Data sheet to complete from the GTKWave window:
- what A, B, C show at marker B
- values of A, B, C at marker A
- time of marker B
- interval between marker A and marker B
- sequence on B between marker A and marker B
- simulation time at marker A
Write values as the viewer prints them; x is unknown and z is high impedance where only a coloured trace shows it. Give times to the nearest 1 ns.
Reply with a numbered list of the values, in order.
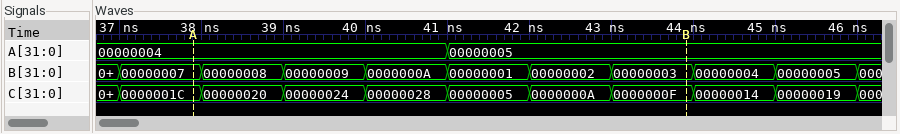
1. A=00000005, B=00000003, C=0000000F
2. A=00000004, B=00000007, C=0000001C
3. 44 ns
4. 6 ns
5. 00000007, 00000008, 00000009, 0000000A, 00000001, 00000002, 00000003
6. 38 ns
